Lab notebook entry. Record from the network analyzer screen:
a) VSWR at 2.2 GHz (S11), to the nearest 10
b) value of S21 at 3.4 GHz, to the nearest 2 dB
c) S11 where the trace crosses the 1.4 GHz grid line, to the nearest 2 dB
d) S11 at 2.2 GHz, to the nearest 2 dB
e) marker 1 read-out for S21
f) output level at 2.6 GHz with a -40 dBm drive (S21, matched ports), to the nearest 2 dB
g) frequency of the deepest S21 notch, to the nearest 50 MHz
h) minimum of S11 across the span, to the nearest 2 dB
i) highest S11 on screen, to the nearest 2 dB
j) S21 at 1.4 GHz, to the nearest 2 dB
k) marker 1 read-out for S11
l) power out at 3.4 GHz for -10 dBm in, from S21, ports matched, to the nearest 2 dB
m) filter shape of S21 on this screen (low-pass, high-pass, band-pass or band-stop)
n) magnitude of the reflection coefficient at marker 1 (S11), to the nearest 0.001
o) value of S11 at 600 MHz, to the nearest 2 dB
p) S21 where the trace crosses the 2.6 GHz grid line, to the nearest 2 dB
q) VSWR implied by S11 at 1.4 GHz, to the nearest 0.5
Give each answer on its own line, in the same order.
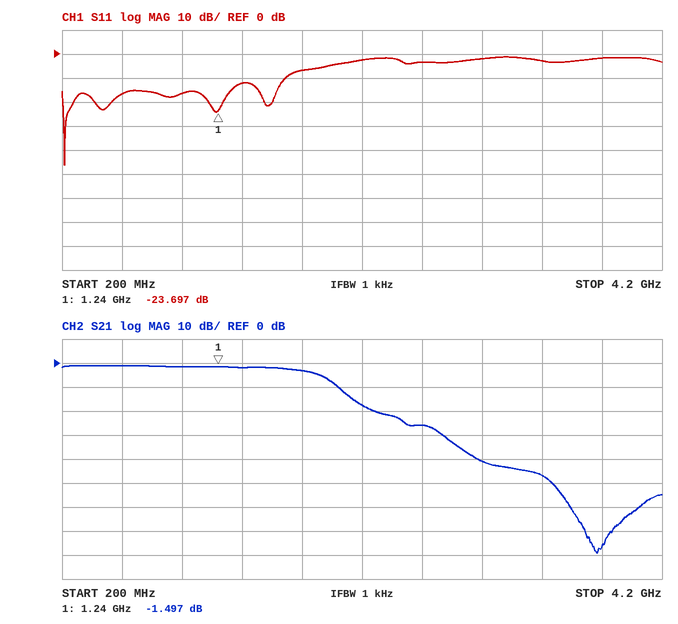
10
-46 dB
-12 dB
-2 dB
-1.497 dB
-66 dBm
3.75 GHz
-46 dB
-2 dB
-2 dB
-23.697 dB
-56 dBm
low-pass
0.065
-16 dB
-26 dB
1.5
